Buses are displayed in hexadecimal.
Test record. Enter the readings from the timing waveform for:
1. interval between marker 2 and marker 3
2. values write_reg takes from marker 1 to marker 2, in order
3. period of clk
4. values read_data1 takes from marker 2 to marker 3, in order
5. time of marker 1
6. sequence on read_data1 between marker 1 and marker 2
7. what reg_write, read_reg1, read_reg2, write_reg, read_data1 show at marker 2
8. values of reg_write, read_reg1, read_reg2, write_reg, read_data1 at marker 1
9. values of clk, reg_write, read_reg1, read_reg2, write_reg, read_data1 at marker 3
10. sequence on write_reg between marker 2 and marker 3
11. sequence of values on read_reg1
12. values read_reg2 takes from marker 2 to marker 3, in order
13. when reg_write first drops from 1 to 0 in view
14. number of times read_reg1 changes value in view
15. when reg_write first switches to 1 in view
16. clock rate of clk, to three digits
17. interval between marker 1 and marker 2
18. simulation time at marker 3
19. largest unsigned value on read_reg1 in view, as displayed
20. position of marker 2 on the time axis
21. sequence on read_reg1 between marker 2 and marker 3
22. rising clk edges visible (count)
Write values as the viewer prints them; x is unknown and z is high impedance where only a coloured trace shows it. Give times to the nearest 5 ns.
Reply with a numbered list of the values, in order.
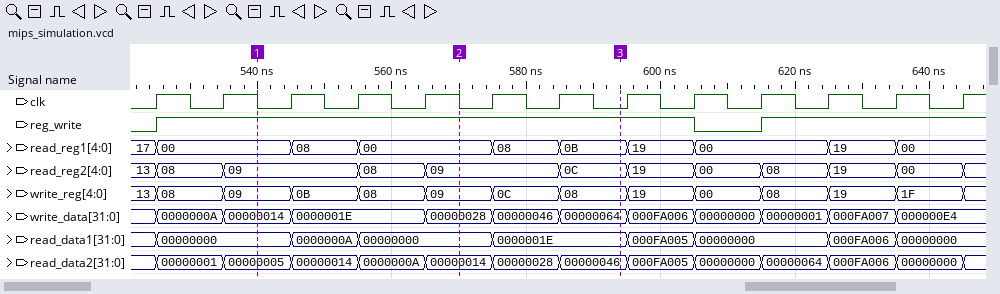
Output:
1. 25 ns
2. 09, 0B, 08, 09
3. 10 ns
4. 00000000, 0000001E
5. 540 ns
6. 00000000, 0000000A, 00000000
7. reg_write=1, read_reg1=00, read_reg2=09, write_reg=09, read_data1=00000000
8. reg_write=1, read_reg1=00, read_reg2=09, write_reg=09, read_data1=00000000
9. clk=0, reg_write=1, read_reg1=0B, read_reg2=0C, write_reg=08, read_data1=0000001E
10. 09, 0C, 08
11. 17, 00, 08, 00, 08, 0B, 19, 00, 19, 00
12. 09, 0C
13. 605 ns
14. 9
15. 525 ns
16. 100 MHz
17. 30 ns
18. 595 ns
19. 19
20. 570 ns
21. 00, 08, 0B
22. 13
